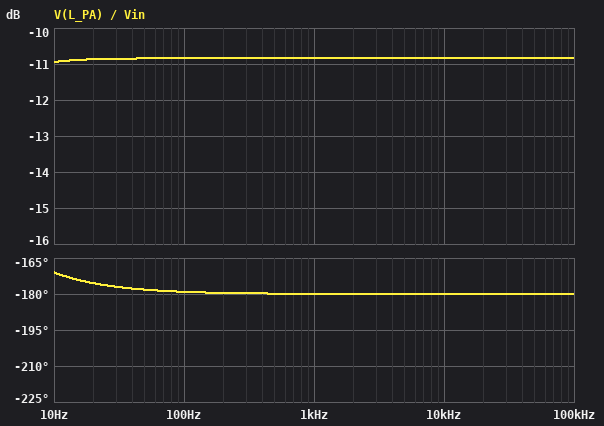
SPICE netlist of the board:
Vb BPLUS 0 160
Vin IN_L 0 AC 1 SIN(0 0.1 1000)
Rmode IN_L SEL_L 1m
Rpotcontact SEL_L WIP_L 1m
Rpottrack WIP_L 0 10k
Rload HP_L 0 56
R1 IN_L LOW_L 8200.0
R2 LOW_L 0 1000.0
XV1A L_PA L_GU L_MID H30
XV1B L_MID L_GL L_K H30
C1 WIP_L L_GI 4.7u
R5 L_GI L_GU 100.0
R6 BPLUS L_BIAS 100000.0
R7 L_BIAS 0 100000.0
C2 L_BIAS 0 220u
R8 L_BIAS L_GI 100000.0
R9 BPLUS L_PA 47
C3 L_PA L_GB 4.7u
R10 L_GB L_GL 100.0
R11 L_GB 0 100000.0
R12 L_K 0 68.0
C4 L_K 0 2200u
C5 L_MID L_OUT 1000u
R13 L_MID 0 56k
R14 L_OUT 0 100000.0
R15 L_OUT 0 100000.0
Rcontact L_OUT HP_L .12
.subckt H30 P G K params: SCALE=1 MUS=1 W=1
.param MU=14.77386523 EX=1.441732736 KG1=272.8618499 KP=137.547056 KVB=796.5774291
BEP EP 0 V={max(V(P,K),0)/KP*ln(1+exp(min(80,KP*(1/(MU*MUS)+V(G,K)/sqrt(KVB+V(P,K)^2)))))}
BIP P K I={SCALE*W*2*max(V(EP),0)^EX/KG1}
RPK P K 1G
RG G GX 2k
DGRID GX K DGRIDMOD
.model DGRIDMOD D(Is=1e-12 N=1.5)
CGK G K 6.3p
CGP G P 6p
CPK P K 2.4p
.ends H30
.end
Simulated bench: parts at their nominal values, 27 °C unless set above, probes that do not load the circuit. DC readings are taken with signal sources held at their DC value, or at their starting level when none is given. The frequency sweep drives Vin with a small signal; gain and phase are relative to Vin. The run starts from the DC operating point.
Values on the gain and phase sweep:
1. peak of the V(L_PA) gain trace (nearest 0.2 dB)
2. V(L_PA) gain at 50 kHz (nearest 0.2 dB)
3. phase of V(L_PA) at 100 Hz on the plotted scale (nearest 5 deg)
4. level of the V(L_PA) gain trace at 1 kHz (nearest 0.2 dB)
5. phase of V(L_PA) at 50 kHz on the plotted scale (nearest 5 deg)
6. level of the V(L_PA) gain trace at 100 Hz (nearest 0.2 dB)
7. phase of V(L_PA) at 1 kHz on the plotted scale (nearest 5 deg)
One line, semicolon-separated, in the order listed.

-10.8 dB; -10.8 dB; -180 deg; -10.8 dB; -180 deg; -10.8 dB; -180 deg
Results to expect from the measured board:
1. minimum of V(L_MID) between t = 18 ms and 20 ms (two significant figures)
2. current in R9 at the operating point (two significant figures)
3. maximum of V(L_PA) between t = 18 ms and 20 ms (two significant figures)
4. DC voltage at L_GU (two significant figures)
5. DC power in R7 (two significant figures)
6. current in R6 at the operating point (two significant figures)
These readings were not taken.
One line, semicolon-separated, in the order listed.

82 V; 38 mA; 160 V; 80 V; 64 mW; 800 µA
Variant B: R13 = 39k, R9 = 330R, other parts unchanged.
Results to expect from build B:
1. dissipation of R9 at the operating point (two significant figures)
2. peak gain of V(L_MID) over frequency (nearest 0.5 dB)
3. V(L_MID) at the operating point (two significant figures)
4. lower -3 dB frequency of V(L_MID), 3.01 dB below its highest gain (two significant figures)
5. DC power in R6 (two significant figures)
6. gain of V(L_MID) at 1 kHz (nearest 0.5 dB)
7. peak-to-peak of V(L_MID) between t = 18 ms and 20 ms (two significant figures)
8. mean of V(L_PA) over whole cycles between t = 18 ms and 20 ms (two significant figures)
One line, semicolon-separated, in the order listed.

480 mW; -2.0 dB; 81 V; 290 mHz; 64 mW; -2.5 dB; 150 mV; 150 V
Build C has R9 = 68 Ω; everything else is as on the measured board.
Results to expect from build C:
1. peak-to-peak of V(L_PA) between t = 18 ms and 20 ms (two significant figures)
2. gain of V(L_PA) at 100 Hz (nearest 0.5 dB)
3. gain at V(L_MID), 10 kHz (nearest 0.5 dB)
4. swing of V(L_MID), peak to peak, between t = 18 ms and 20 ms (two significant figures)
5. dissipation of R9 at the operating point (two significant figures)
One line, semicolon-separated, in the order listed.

74 mV; -8.5 dB; -4.5 dB; 120 mV; 98 mW
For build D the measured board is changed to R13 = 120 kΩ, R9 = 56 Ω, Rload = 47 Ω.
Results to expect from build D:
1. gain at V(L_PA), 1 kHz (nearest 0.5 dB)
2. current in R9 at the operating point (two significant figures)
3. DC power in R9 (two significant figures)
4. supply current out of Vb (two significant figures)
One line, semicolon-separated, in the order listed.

-9.0 dB; 37 mA; 78 mW; 38 mA
